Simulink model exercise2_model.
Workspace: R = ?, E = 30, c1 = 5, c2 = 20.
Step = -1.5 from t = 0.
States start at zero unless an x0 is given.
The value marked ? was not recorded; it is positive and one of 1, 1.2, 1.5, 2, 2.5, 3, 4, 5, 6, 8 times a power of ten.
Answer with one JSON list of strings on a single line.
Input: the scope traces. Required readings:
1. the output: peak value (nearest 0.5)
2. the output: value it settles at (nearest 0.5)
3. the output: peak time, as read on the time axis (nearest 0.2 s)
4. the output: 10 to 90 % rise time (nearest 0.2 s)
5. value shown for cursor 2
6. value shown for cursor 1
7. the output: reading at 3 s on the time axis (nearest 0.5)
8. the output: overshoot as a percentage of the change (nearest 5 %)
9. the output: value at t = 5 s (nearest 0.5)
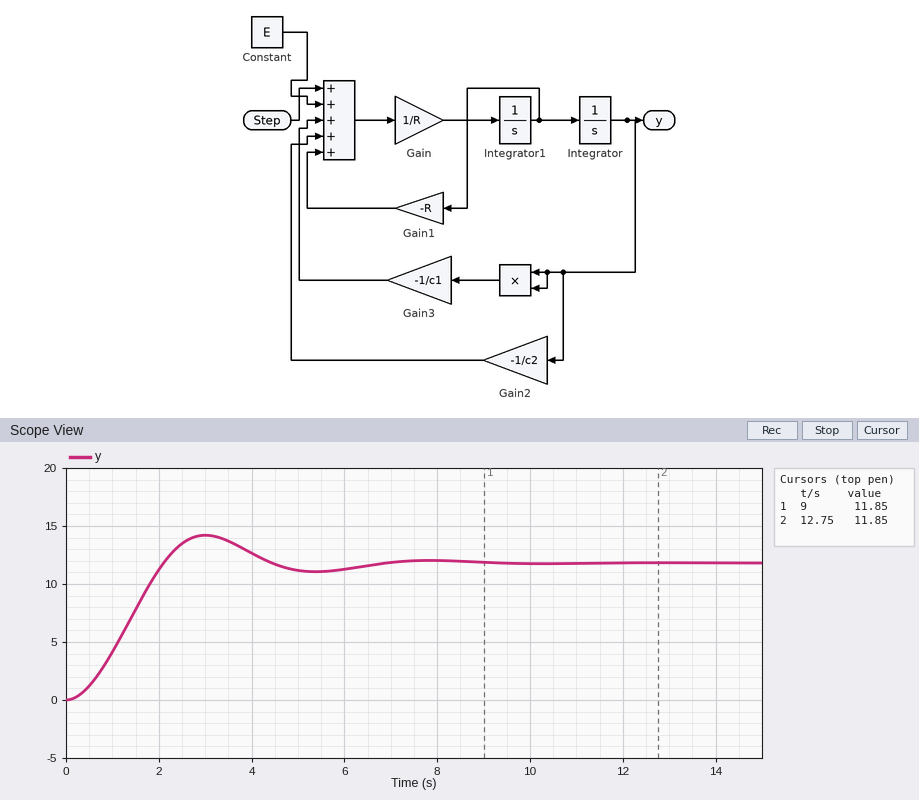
["14.0", "12.0", "3.0 s", "1.4 s", "11.85", "11.85", "14.0", "20 %", "11.0"]
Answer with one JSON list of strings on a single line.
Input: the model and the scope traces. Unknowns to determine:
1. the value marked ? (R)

["2.5"]
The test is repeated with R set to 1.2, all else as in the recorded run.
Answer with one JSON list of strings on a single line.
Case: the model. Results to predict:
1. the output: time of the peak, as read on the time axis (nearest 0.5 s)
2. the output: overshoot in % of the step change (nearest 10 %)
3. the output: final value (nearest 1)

["2.0 s", "30 %", "12"]
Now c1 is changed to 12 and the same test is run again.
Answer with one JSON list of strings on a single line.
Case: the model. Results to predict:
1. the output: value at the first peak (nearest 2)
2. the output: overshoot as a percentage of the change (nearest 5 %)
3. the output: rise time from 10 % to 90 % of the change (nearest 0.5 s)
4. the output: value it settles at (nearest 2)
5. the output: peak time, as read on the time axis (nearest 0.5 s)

["20", "15 %", "2.0 s", "18", "4.0 s"]
